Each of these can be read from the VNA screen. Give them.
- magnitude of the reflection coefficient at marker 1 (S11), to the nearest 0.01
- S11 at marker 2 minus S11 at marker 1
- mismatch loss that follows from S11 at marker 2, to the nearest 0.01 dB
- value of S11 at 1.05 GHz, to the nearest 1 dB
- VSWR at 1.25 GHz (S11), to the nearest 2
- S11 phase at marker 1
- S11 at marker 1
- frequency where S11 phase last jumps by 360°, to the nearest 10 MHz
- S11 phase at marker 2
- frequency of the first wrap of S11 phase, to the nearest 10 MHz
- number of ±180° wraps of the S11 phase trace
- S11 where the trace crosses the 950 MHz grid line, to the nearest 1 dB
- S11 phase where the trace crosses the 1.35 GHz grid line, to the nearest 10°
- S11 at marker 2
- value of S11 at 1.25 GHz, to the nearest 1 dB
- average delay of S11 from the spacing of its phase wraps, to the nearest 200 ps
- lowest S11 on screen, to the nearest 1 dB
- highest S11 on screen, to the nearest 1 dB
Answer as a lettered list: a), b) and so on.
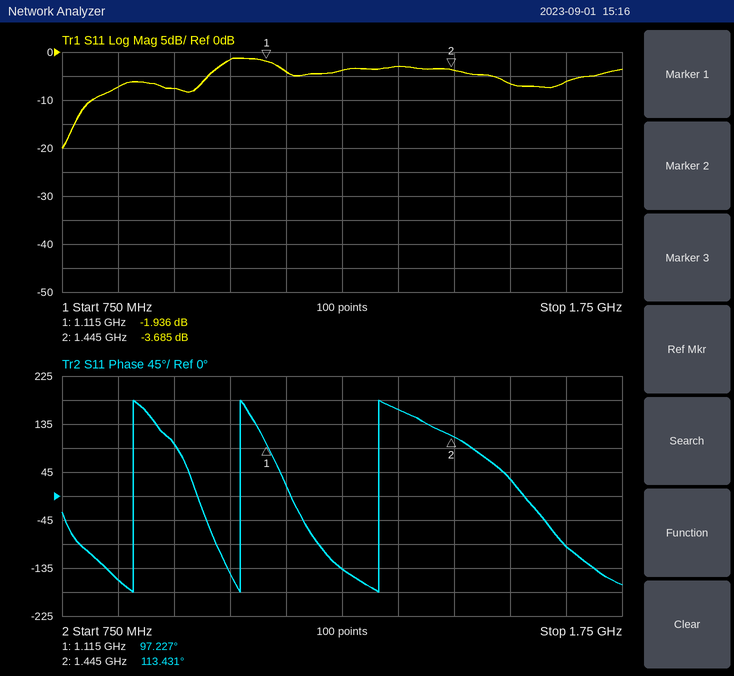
a) 0.80
b) -1.749 dB
c) 2.43 dB
d) -2 dB
e) 4
f) 97.227°
g) -1.936 dB
h) 1.32 GHz
i) 113.431°
j) 880 MHz
k) 3
l) -8 dB
m) 160°
n) -3.685 dB
o) -4 dB
p) 4.6 ns
q) -20 dB
r) -1 dB
